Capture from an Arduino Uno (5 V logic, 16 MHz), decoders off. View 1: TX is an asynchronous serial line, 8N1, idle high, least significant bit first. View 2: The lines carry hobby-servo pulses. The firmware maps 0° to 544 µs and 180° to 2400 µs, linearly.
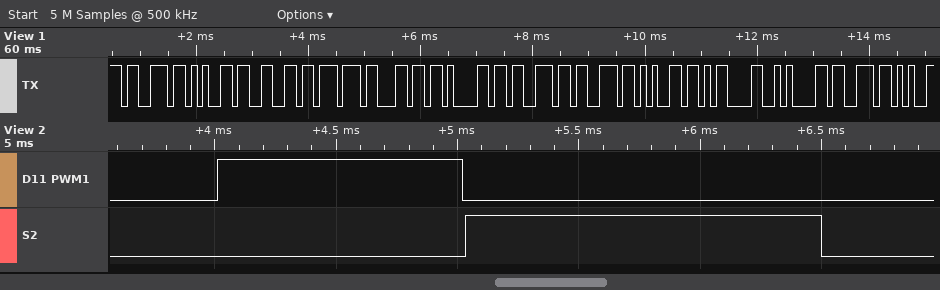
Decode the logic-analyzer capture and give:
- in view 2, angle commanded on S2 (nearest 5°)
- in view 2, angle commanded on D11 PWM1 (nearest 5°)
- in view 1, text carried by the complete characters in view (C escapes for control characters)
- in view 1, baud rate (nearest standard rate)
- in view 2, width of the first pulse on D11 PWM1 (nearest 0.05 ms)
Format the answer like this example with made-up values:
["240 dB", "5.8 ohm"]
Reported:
["90°", "45°", "\"sefwlasse\\r\\ns\"", "9600 baud", "1.00 ms"]
